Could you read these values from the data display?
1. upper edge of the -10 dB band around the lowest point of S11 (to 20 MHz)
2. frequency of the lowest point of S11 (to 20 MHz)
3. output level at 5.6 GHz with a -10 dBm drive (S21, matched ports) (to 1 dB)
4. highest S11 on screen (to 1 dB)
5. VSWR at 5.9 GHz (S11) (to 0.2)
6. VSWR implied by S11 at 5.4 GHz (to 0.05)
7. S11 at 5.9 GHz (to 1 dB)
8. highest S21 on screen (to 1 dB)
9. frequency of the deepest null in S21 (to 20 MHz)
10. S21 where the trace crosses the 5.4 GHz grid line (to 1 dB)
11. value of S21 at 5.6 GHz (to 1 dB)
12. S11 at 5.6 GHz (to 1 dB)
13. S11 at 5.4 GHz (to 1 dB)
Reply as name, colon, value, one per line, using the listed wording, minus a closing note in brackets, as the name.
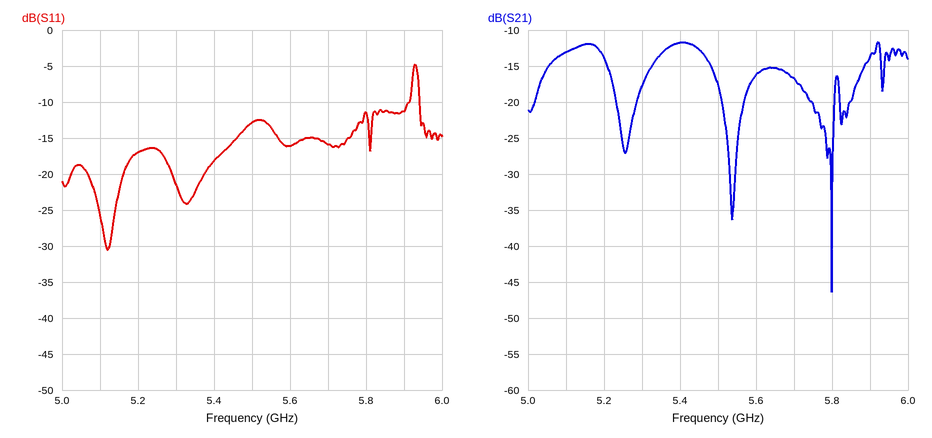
upper edge of the -10 dB band around the lowest point of S11: 5.92 GHz
frequency of the lowest point of S11: 5.12 GHz
output level at 5.6 GHz with a -10 dBm drive (S21, matched ports): -26 dBm
highest S11 on screen: -5 dB
VSWR at 5.9 GHz (S11): 1.8
VSWR implied by S11 at 5.4 GHz: 1.30
S11 at 5.9 GHz: -11 dB
highest S21 on screen: -12 dB
frequency of the deepest null in S21: 5.80 GHz
S21 where the trace crosses the 5.4 GHz grid line: -12 dB
value of S21 at 5.6 GHz: -16 dB
S11 at 5.6 GHz: -16 dB
S11 at 5.4 GHz: -18 dB
